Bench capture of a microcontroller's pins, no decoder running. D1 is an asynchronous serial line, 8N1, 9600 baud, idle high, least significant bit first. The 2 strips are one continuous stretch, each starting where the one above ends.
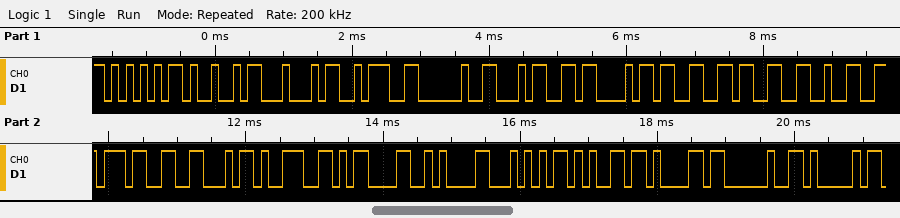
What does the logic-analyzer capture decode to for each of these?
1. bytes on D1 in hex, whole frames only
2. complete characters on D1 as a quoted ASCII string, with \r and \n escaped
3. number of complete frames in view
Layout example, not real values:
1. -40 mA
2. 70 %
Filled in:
1. 55 49 44 3A 20 34 43 33 33 32 37 46 39 0D 0A 54 65 61 20 41
2. "UID: 4C3327F9\r\nTea A"
3. 20
